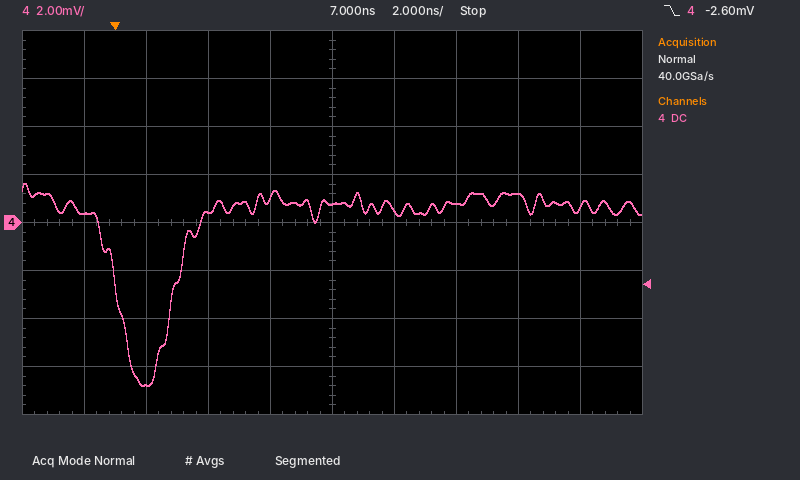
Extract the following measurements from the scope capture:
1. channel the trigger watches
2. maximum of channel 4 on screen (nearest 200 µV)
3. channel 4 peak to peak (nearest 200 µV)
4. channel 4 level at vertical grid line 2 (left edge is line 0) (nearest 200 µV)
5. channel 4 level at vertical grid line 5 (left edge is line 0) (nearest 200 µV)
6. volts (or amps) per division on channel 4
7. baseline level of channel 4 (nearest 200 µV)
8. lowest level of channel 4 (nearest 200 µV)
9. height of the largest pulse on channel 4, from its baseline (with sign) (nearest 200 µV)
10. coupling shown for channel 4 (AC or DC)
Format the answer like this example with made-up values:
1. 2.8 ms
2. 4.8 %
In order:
1. channel 4
2. 1.6 mV
3. 8.4 mV
4. -6.8 mV
5. 800 µV
6. 2 mV
7. 800 µV
8. -6.8 mV
9. -7.6 mV
10. DC
